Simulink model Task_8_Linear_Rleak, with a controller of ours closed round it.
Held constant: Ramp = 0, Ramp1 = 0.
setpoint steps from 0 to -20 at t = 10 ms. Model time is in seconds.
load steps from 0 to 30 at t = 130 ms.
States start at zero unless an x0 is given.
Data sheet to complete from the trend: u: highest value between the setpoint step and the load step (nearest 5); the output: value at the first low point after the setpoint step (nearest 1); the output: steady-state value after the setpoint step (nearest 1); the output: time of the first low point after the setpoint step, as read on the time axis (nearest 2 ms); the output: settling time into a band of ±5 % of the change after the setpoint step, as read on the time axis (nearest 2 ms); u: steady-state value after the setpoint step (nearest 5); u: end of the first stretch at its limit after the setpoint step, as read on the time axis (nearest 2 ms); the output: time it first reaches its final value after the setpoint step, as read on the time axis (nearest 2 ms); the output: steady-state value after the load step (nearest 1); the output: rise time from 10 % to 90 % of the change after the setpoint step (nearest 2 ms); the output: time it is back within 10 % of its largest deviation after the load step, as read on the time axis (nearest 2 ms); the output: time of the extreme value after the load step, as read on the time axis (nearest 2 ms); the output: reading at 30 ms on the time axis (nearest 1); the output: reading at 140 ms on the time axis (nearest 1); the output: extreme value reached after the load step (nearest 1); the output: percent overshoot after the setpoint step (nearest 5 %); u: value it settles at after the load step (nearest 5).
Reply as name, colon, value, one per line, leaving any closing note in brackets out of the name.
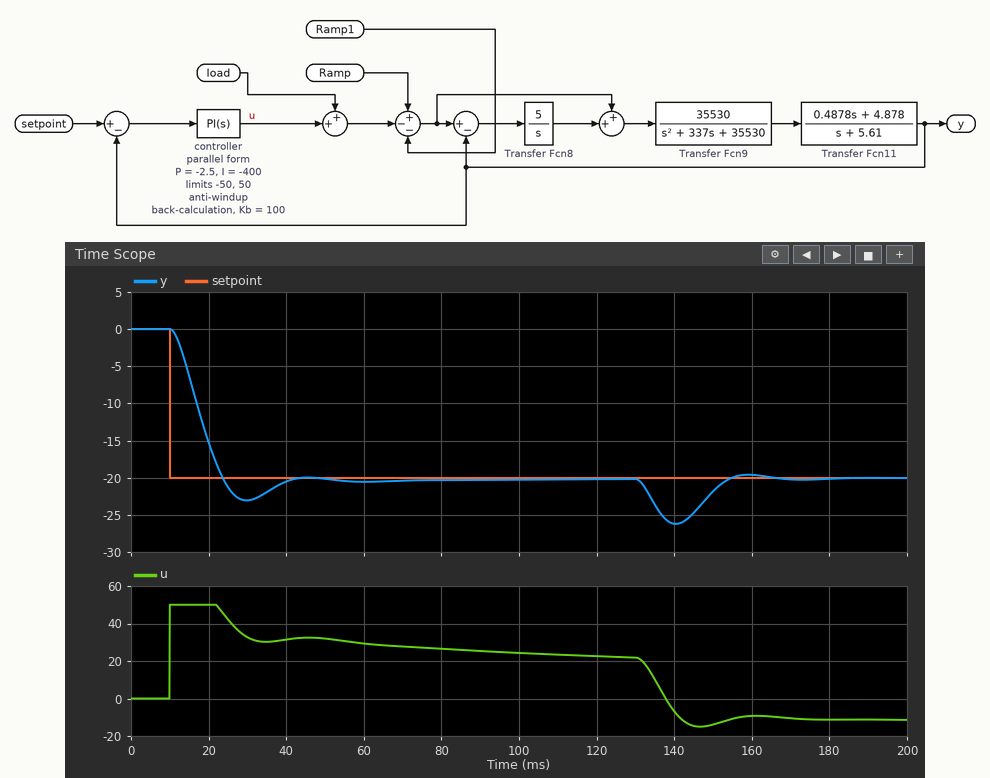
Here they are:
u: highest value between the setpoint step and the load step: 50
the output: value at the first low point after the setpoint step: -23
the output: steady-state value after the setpoint step: -20
the output: time of the first low point after the setpoint step, as read on the time axis: 30 ms
the output: settling time into a band of ±5 % of the change after the setpoint step, as read on the time axis: 38 ms
u: steady-state value after the setpoint step: 20
u: end of the first stretch at its limit after the setpoint step, as read on the time axis: 22 ms
the output: time it first reaches its final value after the setpoint step, as read on the time axis: 24 ms
the output: steady-state value after the load step: -20
the output: rise time from 10 % to 90 % of the change after the setpoint step: 10 ms
the output: time it is back within 10 % of its largest deviation after the load step, as read on the time axis: 152 ms
the output: time of the extreme value after the load step, as read on the time axis: 140 ms
the output: reading at 30 ms on the time axis: -23
the output: reading at 140 ms on the time axis: -26
the output: extreme value reached after the load step: -26
the output: percent overshoot after the setpoint step: 15 %
u: value it settles at after the load step: -10
